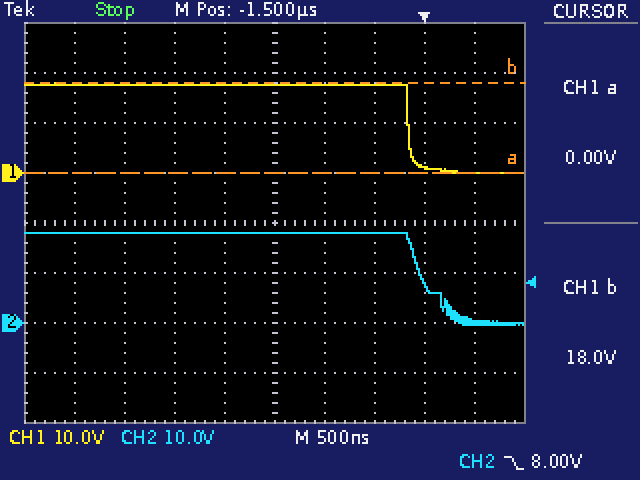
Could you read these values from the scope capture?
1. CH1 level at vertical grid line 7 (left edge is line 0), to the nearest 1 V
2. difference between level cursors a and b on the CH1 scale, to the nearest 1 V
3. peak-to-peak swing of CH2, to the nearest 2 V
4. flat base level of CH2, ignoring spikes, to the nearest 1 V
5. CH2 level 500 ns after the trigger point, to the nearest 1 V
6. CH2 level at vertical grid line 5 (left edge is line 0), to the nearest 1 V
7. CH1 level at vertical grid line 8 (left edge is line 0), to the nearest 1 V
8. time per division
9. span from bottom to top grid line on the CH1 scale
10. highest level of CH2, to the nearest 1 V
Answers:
18 V
18 V
18 V
0 V
0 V
18 V
1 V
500 ns
80 V
18 V
